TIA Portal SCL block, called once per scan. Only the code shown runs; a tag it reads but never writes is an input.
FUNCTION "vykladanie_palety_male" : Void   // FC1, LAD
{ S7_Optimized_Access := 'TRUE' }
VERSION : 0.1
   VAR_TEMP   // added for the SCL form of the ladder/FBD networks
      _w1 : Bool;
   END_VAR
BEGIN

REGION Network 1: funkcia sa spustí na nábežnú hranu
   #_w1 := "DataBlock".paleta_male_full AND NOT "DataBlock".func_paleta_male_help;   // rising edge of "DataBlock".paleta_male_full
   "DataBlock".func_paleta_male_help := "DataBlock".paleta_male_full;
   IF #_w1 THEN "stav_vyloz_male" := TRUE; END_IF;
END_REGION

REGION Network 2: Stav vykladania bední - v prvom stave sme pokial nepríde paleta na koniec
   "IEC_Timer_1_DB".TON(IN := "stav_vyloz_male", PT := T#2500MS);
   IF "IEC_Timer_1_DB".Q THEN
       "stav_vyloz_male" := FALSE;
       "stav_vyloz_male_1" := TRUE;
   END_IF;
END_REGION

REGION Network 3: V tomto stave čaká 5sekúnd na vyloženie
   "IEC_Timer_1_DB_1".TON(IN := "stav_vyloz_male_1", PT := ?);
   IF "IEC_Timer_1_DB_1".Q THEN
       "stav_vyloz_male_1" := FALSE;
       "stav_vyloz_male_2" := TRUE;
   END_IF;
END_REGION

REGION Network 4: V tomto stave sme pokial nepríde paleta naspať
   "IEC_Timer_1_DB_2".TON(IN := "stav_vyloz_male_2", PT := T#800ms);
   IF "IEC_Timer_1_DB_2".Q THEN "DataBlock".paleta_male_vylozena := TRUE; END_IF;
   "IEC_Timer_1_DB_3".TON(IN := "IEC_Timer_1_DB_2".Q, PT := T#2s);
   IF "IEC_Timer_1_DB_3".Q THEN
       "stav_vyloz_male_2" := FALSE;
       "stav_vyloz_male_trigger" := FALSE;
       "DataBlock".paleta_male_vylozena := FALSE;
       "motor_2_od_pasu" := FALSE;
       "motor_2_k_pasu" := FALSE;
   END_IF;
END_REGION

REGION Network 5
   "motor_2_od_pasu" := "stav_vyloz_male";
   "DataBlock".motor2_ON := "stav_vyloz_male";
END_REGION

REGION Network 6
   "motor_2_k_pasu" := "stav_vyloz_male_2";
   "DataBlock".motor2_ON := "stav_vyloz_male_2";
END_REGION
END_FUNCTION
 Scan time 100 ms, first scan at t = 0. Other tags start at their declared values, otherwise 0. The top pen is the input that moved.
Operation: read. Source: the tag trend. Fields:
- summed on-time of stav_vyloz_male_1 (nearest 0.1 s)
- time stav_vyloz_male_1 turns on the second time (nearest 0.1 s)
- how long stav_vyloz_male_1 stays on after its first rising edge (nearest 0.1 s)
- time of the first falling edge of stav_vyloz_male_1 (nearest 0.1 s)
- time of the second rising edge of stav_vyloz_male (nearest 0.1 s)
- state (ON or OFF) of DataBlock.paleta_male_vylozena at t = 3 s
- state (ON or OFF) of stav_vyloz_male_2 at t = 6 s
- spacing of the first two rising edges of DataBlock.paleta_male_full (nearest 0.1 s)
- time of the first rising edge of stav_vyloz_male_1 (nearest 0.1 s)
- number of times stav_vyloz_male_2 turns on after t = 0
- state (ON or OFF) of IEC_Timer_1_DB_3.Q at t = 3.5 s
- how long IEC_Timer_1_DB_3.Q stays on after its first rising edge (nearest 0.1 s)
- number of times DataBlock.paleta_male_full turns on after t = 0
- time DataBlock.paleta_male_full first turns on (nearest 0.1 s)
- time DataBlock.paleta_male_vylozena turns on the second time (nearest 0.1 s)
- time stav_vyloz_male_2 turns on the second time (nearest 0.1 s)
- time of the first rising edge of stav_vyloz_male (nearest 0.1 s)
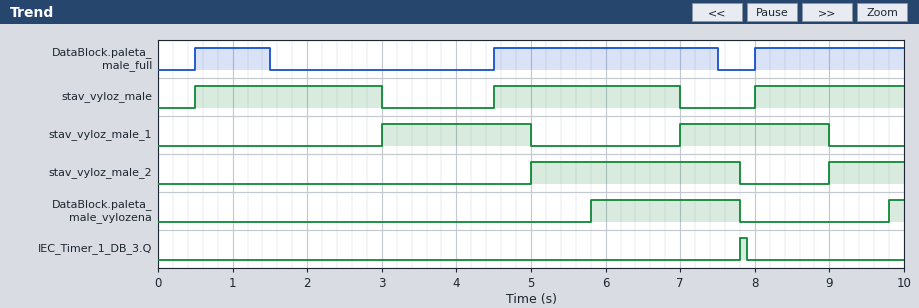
4.0 s
7.0 s
2.0 s
5.0 s
4.5 s
OFF
ON
4.0 s
3.0 s
2
OFF
0.1 s
3
0.5 s
9.8 s
9.0 s
0.5 s
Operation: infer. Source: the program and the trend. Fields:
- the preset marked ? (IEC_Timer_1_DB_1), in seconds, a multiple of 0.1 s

2.0 s
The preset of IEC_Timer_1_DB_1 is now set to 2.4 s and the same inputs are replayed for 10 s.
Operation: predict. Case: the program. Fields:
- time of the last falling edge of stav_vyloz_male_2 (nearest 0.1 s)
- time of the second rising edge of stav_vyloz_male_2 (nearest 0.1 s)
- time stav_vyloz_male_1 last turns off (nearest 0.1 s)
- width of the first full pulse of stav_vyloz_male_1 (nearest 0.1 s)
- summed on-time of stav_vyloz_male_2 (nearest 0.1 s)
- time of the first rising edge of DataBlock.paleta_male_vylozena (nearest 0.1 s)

8.2 s
9.4 s
9.4 s
2.4 s
3.4 s
6.2 s
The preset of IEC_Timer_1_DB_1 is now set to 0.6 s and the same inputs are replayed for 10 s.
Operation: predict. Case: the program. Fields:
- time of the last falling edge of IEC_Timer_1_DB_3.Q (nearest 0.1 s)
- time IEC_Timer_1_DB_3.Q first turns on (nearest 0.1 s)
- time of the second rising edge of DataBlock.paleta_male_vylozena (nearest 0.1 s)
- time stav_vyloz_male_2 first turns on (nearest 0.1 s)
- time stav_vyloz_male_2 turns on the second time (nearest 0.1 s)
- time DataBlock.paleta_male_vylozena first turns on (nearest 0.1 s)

6.5 s
6.4 s
8.4 s
3.6 s
7.6 s
4.4 s
